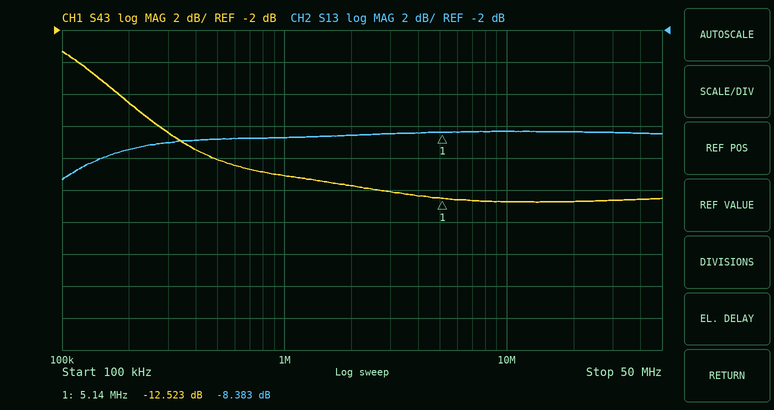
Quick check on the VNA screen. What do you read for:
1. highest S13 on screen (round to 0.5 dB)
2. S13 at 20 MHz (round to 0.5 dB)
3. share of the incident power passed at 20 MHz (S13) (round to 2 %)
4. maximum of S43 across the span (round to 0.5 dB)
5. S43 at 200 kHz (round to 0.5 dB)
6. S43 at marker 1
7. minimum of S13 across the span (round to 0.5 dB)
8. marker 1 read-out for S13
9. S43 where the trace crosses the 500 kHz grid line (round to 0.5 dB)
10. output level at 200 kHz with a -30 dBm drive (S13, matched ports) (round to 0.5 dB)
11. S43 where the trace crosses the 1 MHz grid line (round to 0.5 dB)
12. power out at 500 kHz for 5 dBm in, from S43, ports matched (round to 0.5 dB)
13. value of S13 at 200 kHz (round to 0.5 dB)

-8.5 dB
-8.5 dB
14 %
-3.5 dB
-6.5 dB
-12.523 dB
-11.5 dB
-8.383 dB
-10.0 dB
-39.5 dBm
-11.0 dB
-5.0 dBm
-9.5 dB
